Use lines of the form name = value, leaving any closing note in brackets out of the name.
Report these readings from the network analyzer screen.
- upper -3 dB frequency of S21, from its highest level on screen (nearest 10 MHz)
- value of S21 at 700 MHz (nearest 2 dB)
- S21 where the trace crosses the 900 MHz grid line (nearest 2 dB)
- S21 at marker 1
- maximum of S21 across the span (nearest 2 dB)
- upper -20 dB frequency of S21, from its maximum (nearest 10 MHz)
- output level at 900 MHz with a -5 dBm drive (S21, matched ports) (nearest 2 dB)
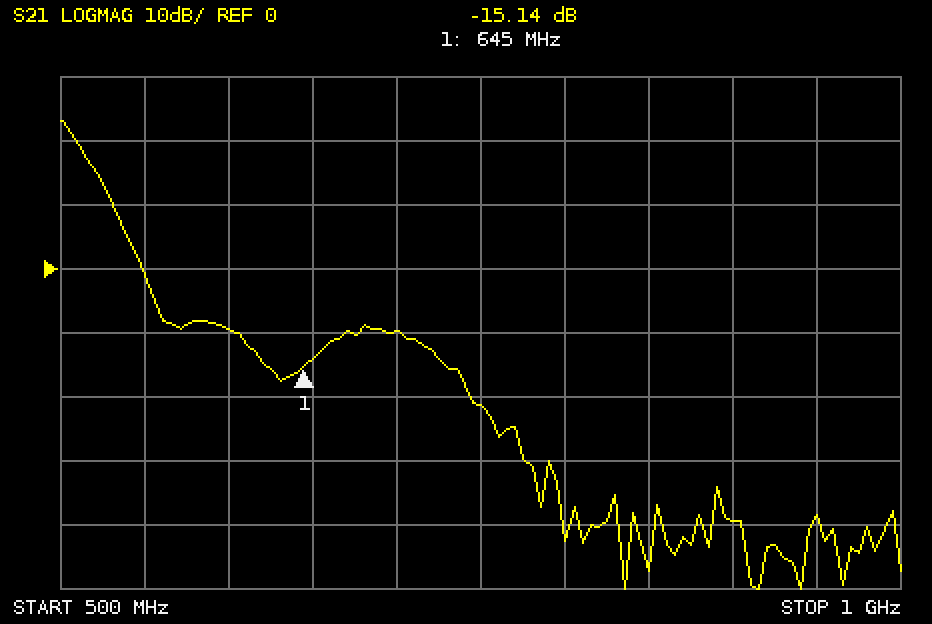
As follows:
upper -3 dB frequency of S21, from its highest level on screen = 510 MHz
value of S21 at 700 MHz = -10 dB
S21 where the trace crosses the 900 MHz grid line = -40 dB
S21 at marker 1 = -15.14 dB
maximum of S21 across the span = 24 dB
upper -20 dB frequency of S21, from its maximum = 540 MHz
output level at 900 MHz with a -5 dBm drive (S21, matched ports) = -44 dBm
